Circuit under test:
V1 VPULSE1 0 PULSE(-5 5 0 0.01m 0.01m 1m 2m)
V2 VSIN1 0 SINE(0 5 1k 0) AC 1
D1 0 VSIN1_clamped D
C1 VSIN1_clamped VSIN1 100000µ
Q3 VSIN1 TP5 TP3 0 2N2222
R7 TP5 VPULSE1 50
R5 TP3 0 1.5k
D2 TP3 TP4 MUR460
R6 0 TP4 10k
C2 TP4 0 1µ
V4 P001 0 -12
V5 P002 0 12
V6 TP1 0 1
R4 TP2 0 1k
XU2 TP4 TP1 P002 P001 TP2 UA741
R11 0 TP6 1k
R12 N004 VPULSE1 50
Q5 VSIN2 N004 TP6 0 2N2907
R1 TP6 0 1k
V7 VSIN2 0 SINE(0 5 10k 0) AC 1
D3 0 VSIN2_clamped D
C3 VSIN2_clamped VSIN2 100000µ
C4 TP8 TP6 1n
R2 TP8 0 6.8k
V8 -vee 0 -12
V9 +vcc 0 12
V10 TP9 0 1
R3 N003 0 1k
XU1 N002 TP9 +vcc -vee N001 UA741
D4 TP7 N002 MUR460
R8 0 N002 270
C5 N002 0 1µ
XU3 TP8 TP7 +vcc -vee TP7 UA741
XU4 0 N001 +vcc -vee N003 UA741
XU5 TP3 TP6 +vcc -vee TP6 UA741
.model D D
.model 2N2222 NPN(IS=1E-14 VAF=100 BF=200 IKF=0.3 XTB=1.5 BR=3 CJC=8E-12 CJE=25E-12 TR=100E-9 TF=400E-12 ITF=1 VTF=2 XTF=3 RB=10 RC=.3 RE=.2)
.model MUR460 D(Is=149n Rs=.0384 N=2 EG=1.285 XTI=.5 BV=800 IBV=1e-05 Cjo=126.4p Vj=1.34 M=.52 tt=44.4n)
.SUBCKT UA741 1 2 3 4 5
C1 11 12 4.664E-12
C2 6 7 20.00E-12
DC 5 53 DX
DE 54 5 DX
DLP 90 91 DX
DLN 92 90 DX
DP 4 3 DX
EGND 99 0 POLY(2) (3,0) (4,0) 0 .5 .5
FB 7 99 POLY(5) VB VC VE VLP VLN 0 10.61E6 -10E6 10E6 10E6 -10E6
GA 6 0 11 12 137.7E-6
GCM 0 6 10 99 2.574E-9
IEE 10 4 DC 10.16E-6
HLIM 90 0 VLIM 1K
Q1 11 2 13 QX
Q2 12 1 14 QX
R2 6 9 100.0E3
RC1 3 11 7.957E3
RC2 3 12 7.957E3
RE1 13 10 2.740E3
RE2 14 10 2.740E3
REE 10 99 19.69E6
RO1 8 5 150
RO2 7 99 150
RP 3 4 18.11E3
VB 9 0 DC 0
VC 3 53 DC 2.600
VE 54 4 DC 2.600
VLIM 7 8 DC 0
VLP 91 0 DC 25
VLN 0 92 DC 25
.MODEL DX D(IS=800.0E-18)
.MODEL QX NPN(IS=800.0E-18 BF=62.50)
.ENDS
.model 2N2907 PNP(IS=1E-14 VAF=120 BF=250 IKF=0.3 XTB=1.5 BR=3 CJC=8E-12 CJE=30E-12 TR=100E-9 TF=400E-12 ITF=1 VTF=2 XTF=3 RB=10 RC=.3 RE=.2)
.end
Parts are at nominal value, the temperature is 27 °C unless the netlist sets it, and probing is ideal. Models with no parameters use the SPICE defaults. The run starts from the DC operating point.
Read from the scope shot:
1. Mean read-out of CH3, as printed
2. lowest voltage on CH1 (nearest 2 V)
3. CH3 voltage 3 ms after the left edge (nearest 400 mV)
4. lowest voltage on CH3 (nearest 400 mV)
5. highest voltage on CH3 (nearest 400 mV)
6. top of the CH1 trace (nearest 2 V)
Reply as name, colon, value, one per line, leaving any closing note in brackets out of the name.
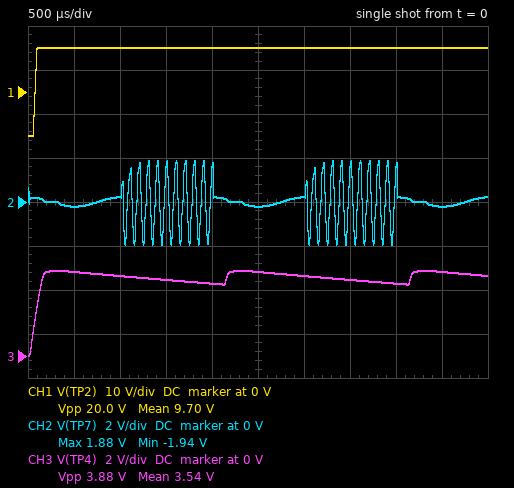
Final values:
Mean read-out of CH3, as printed: 3.54 V
lowest voltage on CH1: -10 V
CH3 voltage 3 ms after the left edge: 3.6 V
lowest voltage on CH3: 0 V
highest voltage on CH3: 4.0 V
top of the CH1 trace: 10 V
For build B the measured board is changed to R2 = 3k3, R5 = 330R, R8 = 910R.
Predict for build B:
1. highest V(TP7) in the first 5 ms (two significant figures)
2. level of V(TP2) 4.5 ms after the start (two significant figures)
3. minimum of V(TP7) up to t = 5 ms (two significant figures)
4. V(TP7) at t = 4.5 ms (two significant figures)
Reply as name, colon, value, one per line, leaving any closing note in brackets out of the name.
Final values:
highest V(TP7) in the first 5 ms: 1.1 V
level of V(TP2) 4.5 ms after the start: 10 V
minimum of V(TP7) up to t = 5 ms: -1.0 V
V(TP7) at t = 4.5 ms: -100 mV
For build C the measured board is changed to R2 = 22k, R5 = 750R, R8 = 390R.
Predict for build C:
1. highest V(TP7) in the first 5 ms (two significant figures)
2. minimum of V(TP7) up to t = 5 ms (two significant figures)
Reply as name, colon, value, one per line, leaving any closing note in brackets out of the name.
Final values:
highest V(TP7) in the first 5 ms: 3.2 V
minimum of V(TP7) up to t = 5 ms: -4.0 V
